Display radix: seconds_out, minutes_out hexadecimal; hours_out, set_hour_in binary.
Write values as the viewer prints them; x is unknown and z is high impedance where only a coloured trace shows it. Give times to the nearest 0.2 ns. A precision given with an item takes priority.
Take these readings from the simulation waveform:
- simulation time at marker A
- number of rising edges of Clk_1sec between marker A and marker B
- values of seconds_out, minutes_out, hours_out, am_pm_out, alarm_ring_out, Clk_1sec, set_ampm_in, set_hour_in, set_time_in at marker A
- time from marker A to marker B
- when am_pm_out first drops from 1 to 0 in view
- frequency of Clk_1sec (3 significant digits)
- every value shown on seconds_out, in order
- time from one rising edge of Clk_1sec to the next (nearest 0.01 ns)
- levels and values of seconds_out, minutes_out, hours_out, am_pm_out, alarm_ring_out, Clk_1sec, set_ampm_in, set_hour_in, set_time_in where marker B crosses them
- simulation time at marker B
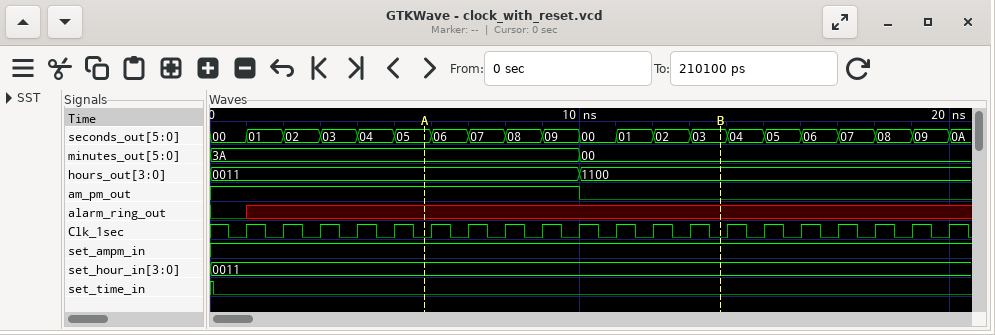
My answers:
5.8 ns
8
seconds_out=05, minutes_out=3A, hours_out=0011, am_pm_out=1, alarm_ring_out=x, Clk_1sec=0, set_ampm_in=1, set_hour_in=0011, set_time_in=0
8 ns
10 ns
1.00 GHz
00, 01, 02, 03, 04, 05, 06, 07, 08, 09, 00, 01, 02, 03, 04, 05, 06, 07, 08, 09, 0A
1 ns
seconds_out=03, minutes_out=00, hours_out=1100, am_pm_out=0, alarm_ring_out=x, Clk_1sec=0, set_ampm_in=1, set_hour_in=0011, set_time_in=0
13.8 ns
